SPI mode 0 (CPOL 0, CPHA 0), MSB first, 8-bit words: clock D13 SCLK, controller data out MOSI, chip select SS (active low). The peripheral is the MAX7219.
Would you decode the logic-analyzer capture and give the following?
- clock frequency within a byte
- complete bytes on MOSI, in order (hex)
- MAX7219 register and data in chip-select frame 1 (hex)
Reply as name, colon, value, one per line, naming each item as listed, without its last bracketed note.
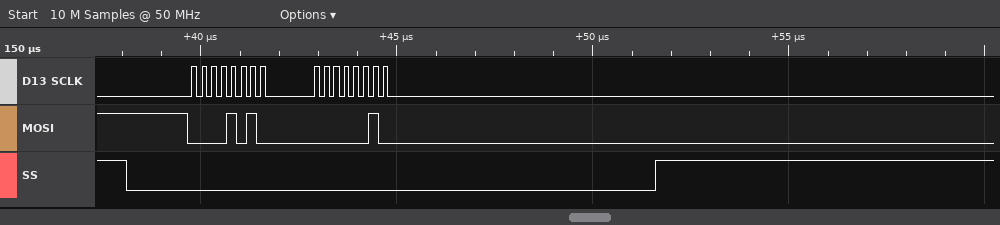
clock frequency within a byte: 4 MHz
complete bytes on MOSI, in order: 0x0A 0x02
MAX7219 register and data in chip-select frame 1: register 0xA, data 0x02
